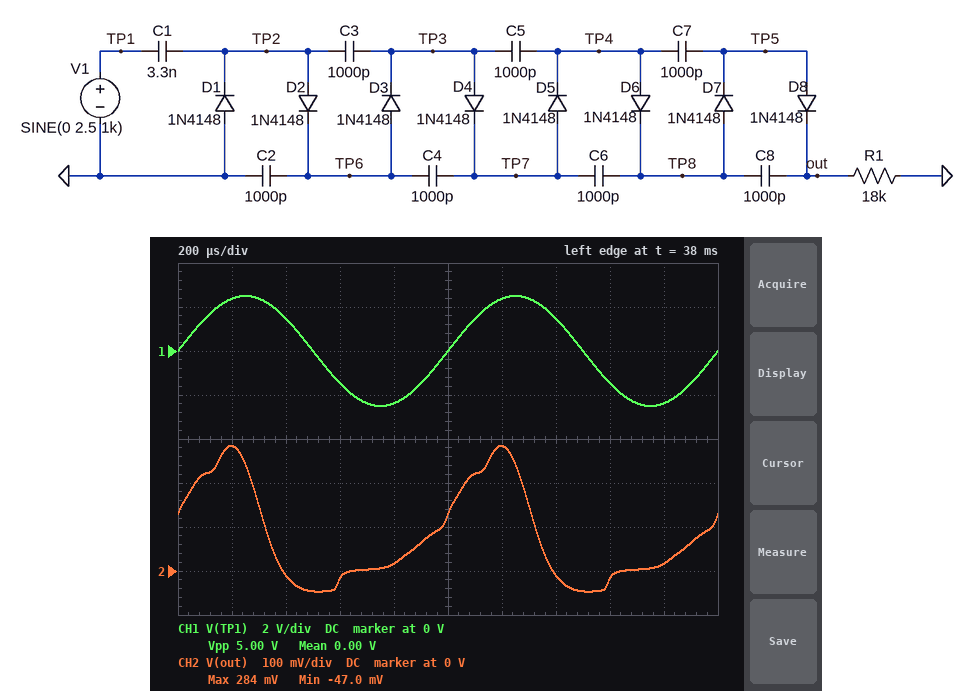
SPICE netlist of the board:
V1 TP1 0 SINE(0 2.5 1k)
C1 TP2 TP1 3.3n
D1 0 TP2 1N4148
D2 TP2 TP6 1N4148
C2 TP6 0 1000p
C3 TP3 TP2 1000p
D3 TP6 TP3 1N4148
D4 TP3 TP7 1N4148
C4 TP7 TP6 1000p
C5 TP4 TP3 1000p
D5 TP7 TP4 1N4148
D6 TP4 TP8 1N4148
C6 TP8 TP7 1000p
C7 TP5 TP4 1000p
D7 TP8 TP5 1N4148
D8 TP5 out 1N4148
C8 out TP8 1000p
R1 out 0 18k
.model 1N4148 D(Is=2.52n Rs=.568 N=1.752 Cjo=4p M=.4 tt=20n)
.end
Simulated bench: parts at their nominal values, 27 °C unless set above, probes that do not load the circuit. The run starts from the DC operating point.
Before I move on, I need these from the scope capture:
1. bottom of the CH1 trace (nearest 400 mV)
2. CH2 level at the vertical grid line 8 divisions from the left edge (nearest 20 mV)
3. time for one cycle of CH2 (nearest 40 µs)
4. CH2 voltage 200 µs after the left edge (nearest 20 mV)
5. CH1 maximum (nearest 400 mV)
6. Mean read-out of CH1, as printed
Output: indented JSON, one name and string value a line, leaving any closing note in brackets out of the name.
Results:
{
  "bottom of the CH1 trace": "-2.4 V",
  "CH2 level at the vertical grid line 8 divisions from the left edge": "-20 mV",
  "time for one cycle of CH2": "1.00 ms",
  "CH2 voltage 200 µs after the left edge": "280 mV",
  "CH1 maximum": "2.4 V",
  "Mean read-out of CH1, as printed": "0.00 V"
}
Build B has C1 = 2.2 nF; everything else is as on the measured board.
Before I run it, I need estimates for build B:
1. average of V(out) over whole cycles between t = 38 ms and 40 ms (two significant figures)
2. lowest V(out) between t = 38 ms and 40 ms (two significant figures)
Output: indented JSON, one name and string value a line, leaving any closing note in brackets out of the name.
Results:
{
  "average of V(out) over whole cycles between t = 38 ms and 40 ms": "52 mV",
  "lowest V(out) between t = 38 ms and 40 ms": "-44 mV"
}
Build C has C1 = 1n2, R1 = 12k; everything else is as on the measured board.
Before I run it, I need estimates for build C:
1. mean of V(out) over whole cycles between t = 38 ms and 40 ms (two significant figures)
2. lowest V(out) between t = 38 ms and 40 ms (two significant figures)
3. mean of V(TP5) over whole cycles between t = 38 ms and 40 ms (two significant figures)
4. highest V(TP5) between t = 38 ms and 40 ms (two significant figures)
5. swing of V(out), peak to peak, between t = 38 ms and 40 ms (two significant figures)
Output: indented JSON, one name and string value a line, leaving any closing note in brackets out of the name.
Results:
{
  "mean of V(out) over whole cycles between t = 38 ms and 40 ms": "18 mV",
  "lowest V(out) between t = 38 ms and 40 ms": "-25 mV",
  "mean of V(TP5) over whole cycles between t = 38 ms and 40 ms": "190 mV",
  "highest V(TP5) between t = 38 ms and 40 ms": "420 mV",
  "swing of V(out), peak to peak, between t = 38 ms and 40 ms": "94 mV"
}
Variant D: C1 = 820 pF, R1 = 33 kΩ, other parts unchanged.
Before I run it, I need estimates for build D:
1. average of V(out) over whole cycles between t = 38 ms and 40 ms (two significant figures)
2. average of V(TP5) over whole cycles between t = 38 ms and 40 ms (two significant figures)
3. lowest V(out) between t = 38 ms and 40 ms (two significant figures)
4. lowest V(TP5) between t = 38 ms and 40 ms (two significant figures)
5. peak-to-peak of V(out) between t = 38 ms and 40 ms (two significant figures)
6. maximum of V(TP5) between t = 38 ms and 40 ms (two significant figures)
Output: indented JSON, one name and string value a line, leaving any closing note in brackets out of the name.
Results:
{
  "average of V(out) over whole cycles between t = 38 ms and 40 ms": "33 mV",
  "average of V(TP5) over whole cycles between t = 38 ms and 40 ms": "200 mV",
  "lowest V(out) between t = 38 ms and 40 ms": "-59 mV",
  "lowest V(TP5) between t = 38 ms and 40 ms": "-130 mV",
  "peak-to-peak of V(out) between t = 38 ms and 40 ms": "190 mV",
  "maximum of V(TP5) between t = 38 ms and 40 ms": "450 mV"
}
